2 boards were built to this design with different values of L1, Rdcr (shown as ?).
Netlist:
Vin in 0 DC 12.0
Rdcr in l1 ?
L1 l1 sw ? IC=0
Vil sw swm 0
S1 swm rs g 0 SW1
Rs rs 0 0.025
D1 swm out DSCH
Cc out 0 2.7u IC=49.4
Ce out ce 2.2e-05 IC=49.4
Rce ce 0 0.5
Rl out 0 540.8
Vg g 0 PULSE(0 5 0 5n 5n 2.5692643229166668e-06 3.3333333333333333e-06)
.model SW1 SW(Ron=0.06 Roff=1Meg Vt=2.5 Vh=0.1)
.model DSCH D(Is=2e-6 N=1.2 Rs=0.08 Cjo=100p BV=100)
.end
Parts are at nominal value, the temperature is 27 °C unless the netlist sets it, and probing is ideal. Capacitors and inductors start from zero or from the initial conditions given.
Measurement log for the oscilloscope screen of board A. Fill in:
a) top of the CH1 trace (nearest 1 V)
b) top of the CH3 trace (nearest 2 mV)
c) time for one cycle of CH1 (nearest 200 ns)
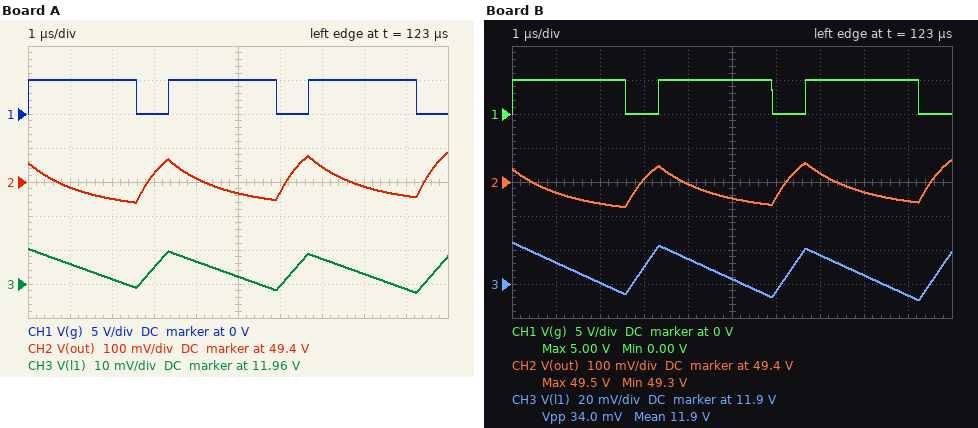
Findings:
5 V
11.970 V
3.4 µs
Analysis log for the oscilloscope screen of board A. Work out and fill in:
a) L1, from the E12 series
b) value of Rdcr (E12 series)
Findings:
150 µH
0.056 Ω
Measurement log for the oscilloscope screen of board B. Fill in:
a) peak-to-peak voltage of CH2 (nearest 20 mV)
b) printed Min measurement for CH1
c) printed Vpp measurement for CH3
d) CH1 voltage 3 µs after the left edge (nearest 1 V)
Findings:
140 mV
0.00 V
34.0 mV
0 V
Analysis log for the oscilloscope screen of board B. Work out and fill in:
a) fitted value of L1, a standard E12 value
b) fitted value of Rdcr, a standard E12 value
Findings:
150 µH
0.15 Ω
